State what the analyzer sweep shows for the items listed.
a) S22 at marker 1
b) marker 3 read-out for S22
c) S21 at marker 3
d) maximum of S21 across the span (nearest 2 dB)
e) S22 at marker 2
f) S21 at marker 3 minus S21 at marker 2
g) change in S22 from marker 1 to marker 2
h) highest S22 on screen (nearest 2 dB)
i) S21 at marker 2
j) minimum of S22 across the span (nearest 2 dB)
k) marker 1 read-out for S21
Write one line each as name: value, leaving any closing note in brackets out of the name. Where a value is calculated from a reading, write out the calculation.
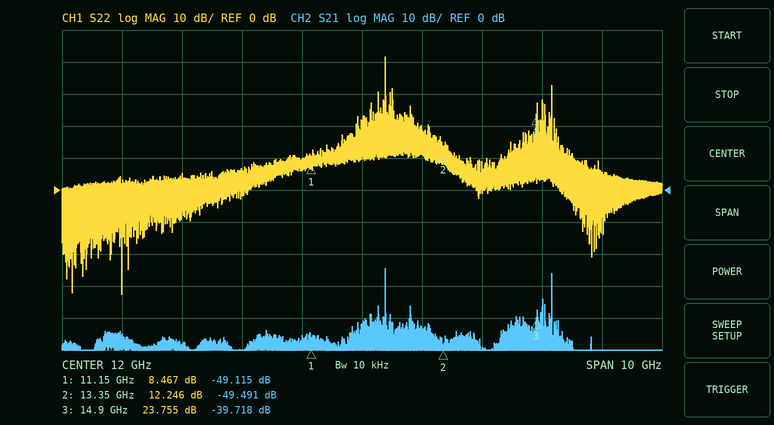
S22 at marker 1: 8.467 dB
marker 3 read-out for S22: 23.755 dB
S21 at marker 3: -39.718 dB
maximum of S21 across the span: -24 dB
S22 at marker 2: 12.246 dB
S21 at marker 3 minus S21 at marker 2: -39.718 − (-49.491) = 9.773 dB
change in S22 from marker 1 to marker 2: 12.246 − (8.467) = 3.779 dB
highest S22 on screen: 42 dB
S21 at marker 2: -49.491 dB
minimum of S22 across the span: -32 dB
marker 1 read-out for S21: -49.115 dB
